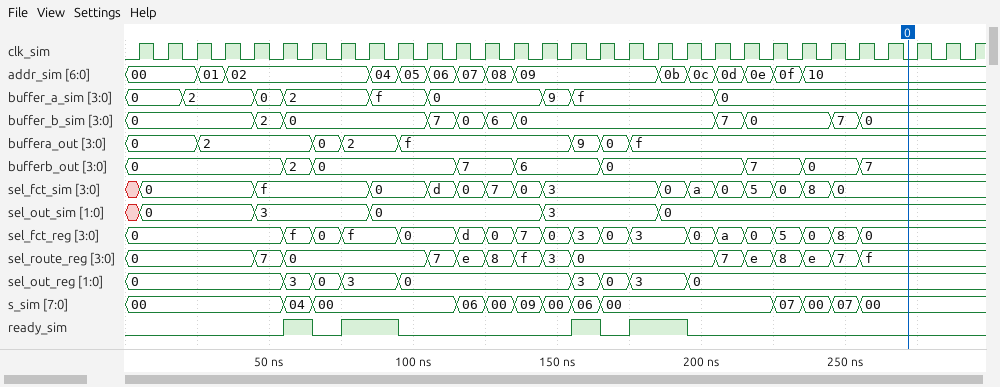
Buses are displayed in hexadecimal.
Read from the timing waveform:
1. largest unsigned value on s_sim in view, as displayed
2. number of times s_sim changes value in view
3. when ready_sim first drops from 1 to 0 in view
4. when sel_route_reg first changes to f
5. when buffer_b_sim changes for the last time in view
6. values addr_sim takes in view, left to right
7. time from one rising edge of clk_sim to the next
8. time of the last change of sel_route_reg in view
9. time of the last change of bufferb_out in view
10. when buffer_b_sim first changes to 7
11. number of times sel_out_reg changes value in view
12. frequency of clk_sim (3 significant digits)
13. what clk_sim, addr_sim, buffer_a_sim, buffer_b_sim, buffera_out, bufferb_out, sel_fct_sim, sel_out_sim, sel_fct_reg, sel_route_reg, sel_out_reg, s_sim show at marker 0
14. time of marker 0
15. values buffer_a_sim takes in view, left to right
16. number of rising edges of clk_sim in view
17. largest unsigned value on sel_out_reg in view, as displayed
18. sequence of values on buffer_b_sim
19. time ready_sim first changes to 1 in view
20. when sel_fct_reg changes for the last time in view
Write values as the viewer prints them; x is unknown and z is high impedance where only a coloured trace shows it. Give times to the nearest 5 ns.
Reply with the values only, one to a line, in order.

09
12
65 ns
135 ns
255 ns
00, 01, 02, 04, 05, 06, 07, 08, 09, 0b, 0c, 0d, 0e, 0f, 10
10 ns
255 ns
255 ns
105 ns
8
100 MHz
clk_sim=0, addr_sim=10, buffer_a_sim=0, buffer_b_sim=0, buffera_out=f, bufferb_out=7, sel_fct_sim=0, sel_out_sim=0, sel_fct_reg=0, sel_route_reg=f, sel_out_reg=0, s_sim=00
270 ns
0, 2, 0, 2, f, 0, 9, f, 0
30
3
0, 2, 0, 7, 0, 6, 0, 7, 0, 7, 0
55 ns
255 ns
